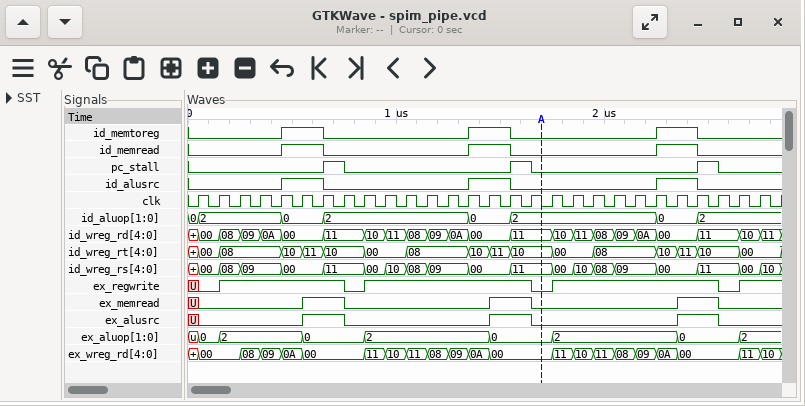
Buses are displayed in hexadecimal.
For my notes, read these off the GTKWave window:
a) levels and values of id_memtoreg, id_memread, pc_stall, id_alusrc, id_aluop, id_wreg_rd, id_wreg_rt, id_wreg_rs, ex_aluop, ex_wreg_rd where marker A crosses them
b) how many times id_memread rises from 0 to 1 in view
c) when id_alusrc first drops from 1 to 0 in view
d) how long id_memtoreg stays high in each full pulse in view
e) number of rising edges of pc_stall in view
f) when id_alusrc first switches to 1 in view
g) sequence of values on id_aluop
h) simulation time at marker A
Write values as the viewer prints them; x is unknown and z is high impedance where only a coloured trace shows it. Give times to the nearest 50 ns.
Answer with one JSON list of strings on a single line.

["id_memtoreg=0, id_memread=0, pc_stall=0, id_alusrc=0, id_aluop=2, id_wreg_rd=11, id_wreg_rt=10, id_wreg_rs=11, ex_aluop=0, ex_wreg_rd=00", "3", "650 ns", "200 ns, 200 ns, 200 ns", "3", "450 ns", "0, 2, 0, 2, 0, 2, 0, 2", "1700 ns"]
